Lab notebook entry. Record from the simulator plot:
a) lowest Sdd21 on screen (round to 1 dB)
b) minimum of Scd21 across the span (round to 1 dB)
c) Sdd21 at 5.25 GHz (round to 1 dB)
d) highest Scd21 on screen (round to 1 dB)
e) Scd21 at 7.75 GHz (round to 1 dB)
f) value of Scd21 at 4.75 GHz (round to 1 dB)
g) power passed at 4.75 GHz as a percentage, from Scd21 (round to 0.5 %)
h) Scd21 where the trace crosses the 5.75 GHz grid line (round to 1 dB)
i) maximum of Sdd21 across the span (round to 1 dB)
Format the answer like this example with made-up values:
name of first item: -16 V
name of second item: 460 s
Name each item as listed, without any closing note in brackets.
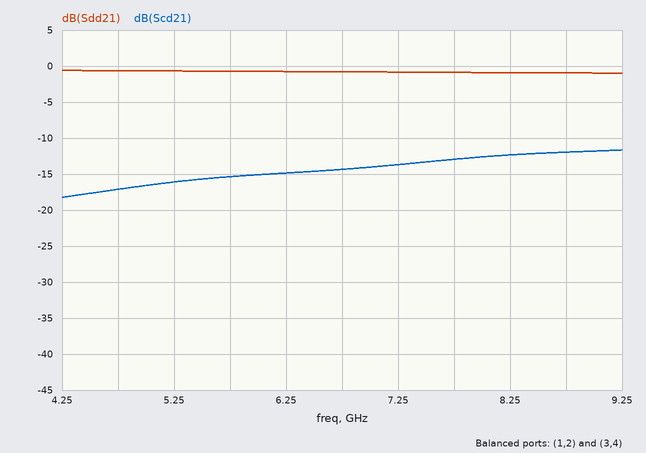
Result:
lowest Sdd21 on screen: -1 dB
minimum of Scd21 across the span: -18 dB
Sdd21 at 5.25 GHz: -1 dB
highest Scd21 on screen: -12 dB
Scd21 at 7.75 GHz: -13 dB
value of Scd21 at 4.75 GHz: -17 dB
power passed at 4.75 GHz as a percentage, from Scd21: 2.0 %
Scd21 where the trace crosses the 5.75 GHz grid line: -15 dB
maximum of Sdd21 across the span: -1 dB
